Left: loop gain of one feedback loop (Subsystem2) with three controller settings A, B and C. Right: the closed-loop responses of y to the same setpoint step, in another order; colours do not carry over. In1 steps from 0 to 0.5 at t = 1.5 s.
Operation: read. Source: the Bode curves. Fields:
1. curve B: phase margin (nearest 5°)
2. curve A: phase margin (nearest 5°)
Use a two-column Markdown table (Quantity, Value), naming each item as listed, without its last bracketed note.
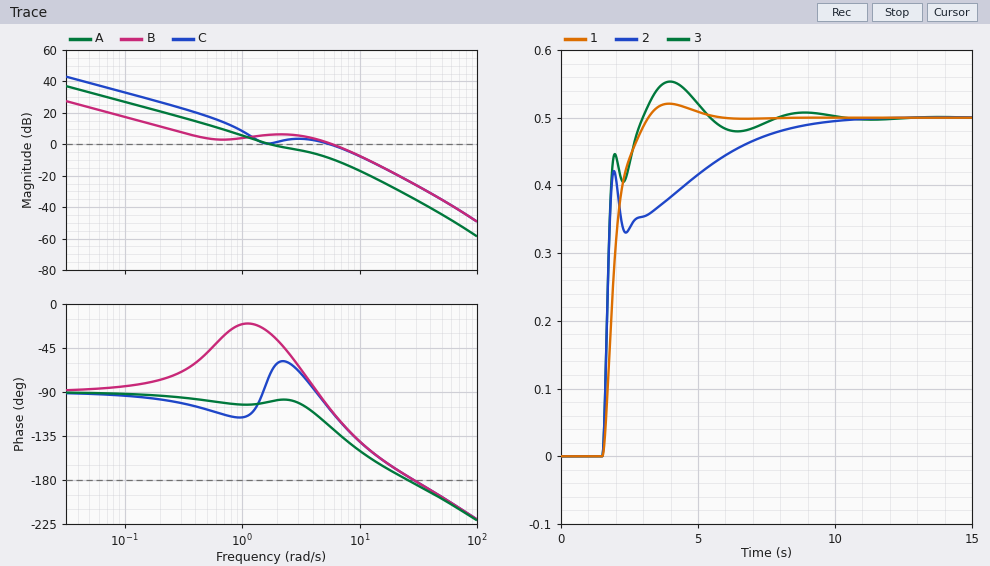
| Quantity | Value |
|---|---|
| curve B: phase margin | 70° |
| curve A: phase margin | 80° |
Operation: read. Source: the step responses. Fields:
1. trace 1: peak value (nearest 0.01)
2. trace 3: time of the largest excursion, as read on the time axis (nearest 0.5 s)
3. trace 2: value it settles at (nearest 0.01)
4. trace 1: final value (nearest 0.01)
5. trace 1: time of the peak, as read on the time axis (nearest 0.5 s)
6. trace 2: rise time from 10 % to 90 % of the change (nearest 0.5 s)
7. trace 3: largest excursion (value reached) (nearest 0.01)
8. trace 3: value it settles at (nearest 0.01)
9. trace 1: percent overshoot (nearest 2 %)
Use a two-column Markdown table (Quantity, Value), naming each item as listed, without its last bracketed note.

| Quantity | Value |
|---|---|
| trace 1: peak value | 0.52 |
| trace 3: time of the largest excursion, as read on the time axis | 4.0 s |
| trace 2: value it settles at | 0.50 |
| trace 1: final value | 0.50 |
| trace 1: time of the peak, as read on the time axis | 4.0 s |
| trace 2: rise time from 10 % to 90 % of the change | 4.5 s |
| trace 3: largest excursion (value reached) | 0.55 |
| trace 3: value it settles at | 0.50 |
| trace 1: percent overshoot | 4 % |
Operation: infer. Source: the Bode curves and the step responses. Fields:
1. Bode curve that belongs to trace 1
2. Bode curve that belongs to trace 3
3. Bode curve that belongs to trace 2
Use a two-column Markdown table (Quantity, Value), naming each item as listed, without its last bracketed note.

| Quantity | Value |
|---|---|
| Bode curve that belongs to trace 1 | A |
| Bode curve that belongs to trace 3 | C |
| Bode curve that belongs to trace 2 | B |
